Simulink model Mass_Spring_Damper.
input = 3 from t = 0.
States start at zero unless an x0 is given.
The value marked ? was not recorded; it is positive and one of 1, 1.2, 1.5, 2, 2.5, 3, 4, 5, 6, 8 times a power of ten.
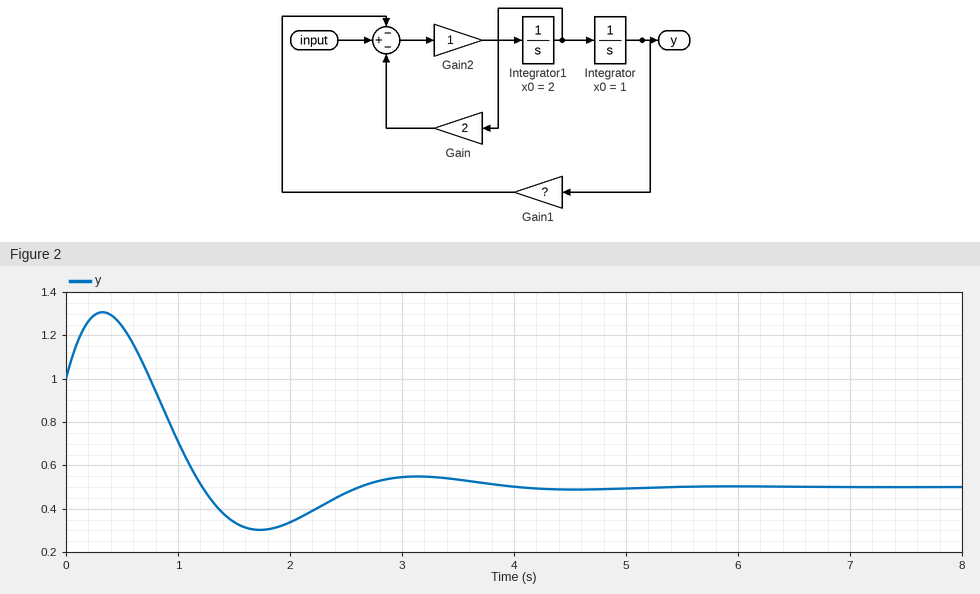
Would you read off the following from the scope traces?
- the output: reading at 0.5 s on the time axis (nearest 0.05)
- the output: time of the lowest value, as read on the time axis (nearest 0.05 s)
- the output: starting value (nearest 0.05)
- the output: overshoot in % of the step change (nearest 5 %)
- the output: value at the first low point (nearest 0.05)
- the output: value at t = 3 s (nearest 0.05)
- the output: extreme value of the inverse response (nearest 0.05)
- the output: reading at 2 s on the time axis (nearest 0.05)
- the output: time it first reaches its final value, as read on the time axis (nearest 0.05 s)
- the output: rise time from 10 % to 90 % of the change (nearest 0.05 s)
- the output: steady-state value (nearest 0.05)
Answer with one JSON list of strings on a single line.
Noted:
["1.25", "1.75 s", "1.00", "40 %", "0.30", "0.55", "1.30", "0.35", "1.20 s", "0.35 s", "0.50"]
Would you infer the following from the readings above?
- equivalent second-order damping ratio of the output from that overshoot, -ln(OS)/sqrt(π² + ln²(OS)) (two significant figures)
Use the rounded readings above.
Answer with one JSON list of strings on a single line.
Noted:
["0.28"]
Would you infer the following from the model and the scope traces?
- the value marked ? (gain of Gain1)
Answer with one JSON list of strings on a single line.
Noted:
["6"]
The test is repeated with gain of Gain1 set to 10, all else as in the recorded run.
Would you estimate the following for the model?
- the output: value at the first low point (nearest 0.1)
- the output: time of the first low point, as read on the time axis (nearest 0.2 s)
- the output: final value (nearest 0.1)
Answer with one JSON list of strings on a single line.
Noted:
["0.0", "1.2 s", "0.3"]
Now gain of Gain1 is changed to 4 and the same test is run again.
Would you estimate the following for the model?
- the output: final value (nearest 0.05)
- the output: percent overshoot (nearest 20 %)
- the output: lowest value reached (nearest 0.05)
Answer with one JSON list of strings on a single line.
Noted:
["0.75", "40 %", "0.65"]
